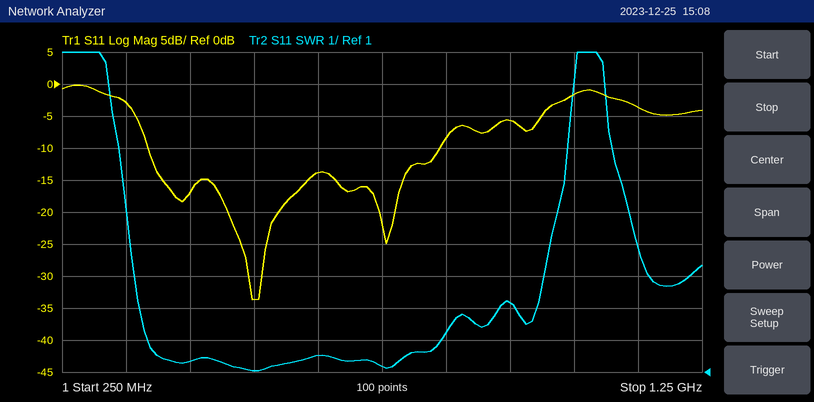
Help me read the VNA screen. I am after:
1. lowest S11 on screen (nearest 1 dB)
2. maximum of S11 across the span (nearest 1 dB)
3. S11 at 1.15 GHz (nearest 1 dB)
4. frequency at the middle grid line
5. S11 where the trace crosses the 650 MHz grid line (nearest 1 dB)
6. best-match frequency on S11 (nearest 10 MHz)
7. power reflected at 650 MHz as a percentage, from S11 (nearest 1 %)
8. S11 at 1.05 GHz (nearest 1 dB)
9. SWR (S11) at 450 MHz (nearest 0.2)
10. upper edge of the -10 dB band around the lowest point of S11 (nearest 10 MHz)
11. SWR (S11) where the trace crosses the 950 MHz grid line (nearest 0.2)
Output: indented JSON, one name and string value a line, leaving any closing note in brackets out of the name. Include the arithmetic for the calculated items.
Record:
{
  "lowest S11 on screen": "-34 dB",
  "maximum of S11 across the span": "0 dB",
  "S11 at 1.15 GHz": "-4 dB",
  "frequency at the middle grid line": "750 MHz",
  "S11 where the trace crosses the 650 MHz grid line": "-14 dB",
  "best-match frequency on S11": "550 MHz",
  "power reflected at 650 MHz as a percentage, from S11": "10^(-14/10) ≈ 4 %",
  "S11 at 1.05 GHz": "-2 dB",
  "SWR (S11) at 450 MHz": "1.4",
  "upper edge of the -10 dB band around the lowest point of S11": "840 MHz",
  "SWR (S11) where the trace crosses the 950 MHz grid line": "3.2"
}
